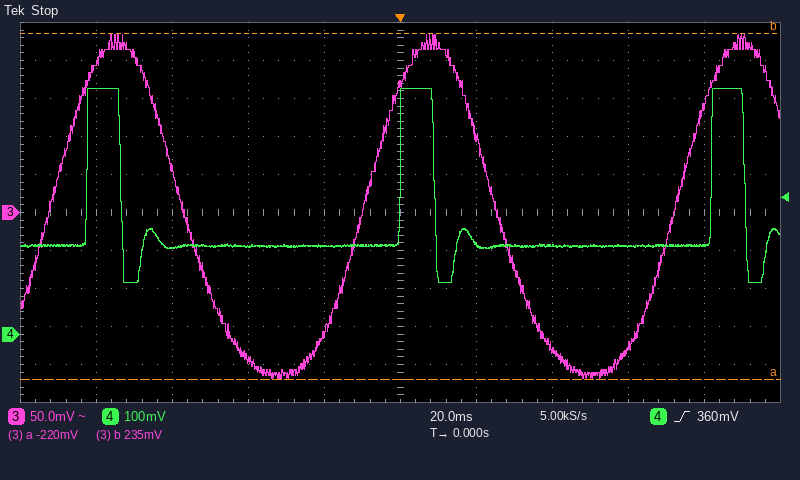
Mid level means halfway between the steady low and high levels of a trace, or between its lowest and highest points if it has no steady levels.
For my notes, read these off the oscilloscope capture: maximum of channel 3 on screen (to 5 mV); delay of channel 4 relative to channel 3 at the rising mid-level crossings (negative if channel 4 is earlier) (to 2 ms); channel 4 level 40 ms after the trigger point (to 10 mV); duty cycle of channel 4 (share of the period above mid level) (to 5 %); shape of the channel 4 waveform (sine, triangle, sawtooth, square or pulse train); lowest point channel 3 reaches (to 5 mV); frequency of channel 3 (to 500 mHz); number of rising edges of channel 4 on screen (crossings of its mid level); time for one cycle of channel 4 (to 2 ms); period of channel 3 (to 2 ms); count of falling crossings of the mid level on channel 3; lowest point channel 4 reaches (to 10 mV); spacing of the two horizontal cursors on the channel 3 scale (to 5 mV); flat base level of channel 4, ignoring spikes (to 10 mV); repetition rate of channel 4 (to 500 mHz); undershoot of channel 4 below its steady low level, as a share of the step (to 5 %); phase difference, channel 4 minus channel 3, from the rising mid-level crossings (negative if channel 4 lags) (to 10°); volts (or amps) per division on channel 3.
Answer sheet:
235 mV
+10 ms
230 mV
10 %
pulse train
-220 mV
12.0 Hz
3
82 ms
82 ms
2
140 mV
455 mV
230 mV
12.0 Hz
25 %
-40°
50 mV
